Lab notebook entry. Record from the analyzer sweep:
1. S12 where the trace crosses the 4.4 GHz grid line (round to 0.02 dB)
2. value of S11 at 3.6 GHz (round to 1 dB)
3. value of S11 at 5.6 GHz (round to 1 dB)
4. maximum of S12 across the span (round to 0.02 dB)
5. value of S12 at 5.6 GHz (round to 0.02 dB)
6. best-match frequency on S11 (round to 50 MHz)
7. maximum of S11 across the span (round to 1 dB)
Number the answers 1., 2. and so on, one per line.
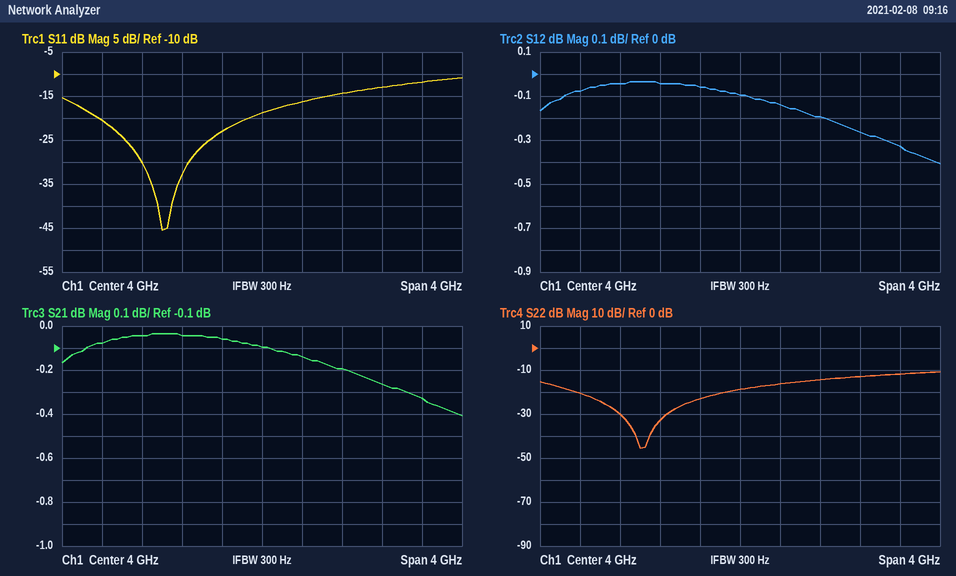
1. -0.14 dB
2. -23 dB
3. -12 dB
4. -0.04 dB
5. -0.32 dB
6. 3.00 GHz
7. -11 dB
